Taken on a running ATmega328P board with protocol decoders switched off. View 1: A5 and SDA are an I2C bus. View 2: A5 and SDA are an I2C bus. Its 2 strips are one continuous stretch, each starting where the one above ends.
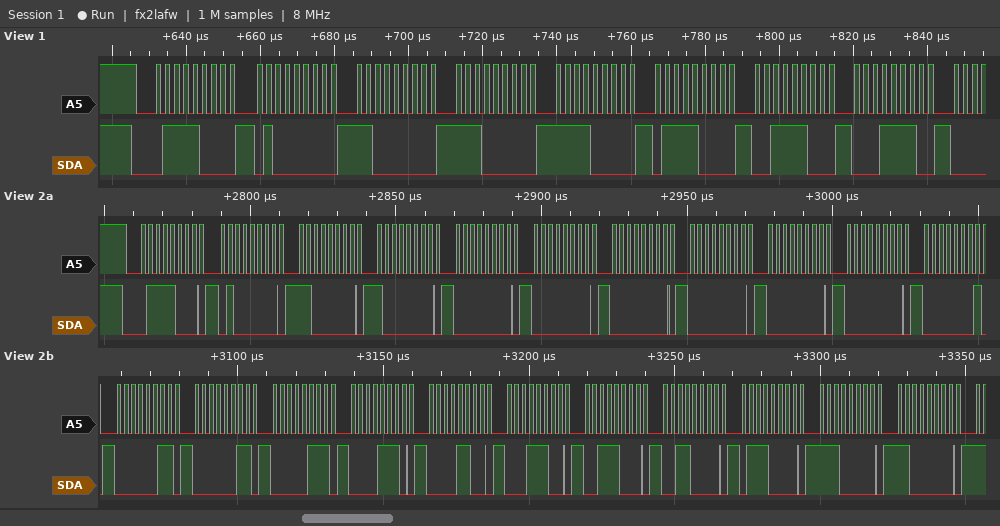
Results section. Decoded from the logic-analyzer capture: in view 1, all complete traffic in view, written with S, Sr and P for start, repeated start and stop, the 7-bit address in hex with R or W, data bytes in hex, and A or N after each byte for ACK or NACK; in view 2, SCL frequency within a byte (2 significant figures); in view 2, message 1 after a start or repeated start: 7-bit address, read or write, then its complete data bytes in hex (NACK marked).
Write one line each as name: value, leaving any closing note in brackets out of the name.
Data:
in view 1, all complete traffic in view, written with S, Sr and P for start, repeated start and stop, the 7-bit address in hex with R or W, data bytes in hex, and A or N after each byte for ACK or NACK: S 3CW A 40 A C0 A E0 A F0 A 78 A 3C A 1E A
in view 2, SCL frequency within a byte: 400 kHz
in view 2, message 1 after a start or repeated start: 7-bit address, read or write, then its complete data bytes in hex: 0x3C write: 40 C0 80 00 00 00 00 00 00 01 03 03 07 0E 0C 1C 38 30 70 E0 C0
